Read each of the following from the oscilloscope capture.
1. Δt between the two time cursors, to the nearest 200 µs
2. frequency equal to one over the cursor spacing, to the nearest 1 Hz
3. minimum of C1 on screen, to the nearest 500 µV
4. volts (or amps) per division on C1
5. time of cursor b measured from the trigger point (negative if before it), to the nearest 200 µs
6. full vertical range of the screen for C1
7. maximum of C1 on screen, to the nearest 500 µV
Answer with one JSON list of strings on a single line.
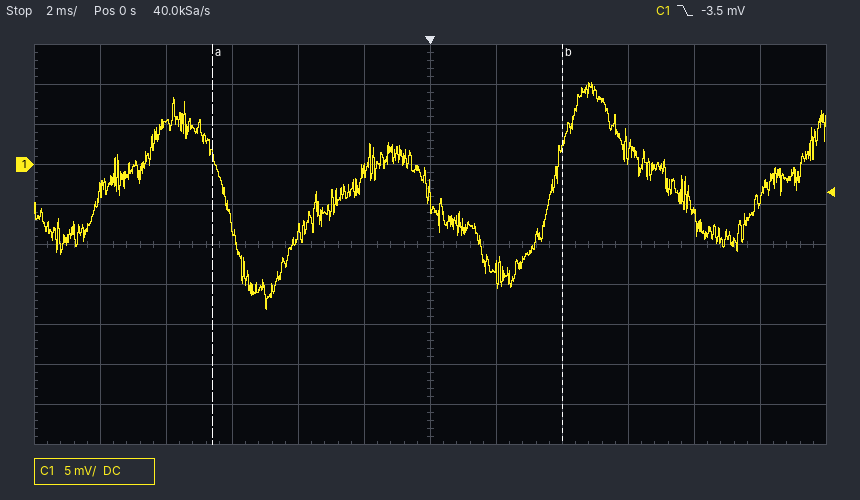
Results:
["10.6 ms", "94 Hz", "-18.0 mV", "5 mV", "+4.0 ms", "50 mV", "10.0 mV"]
